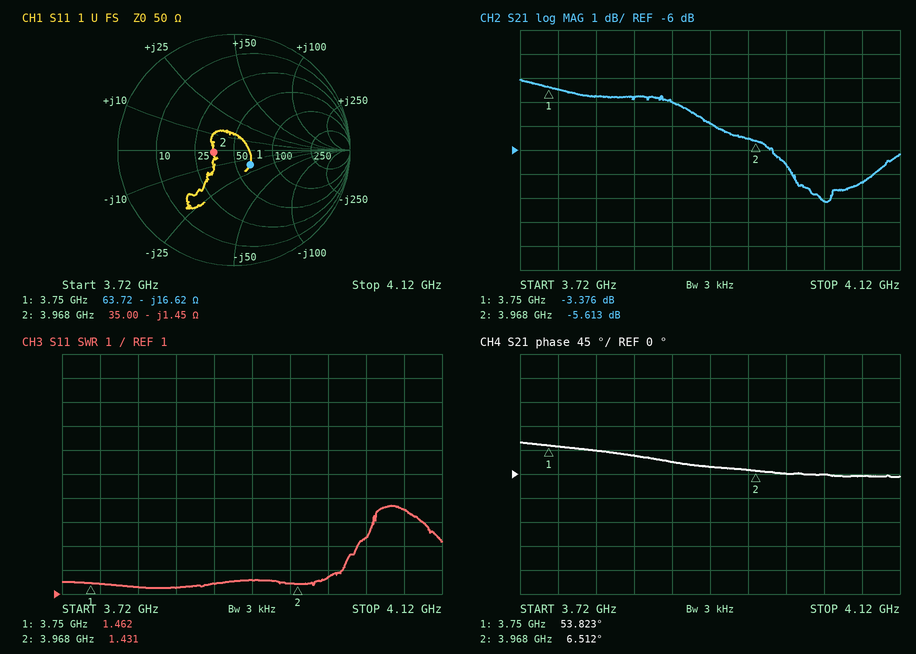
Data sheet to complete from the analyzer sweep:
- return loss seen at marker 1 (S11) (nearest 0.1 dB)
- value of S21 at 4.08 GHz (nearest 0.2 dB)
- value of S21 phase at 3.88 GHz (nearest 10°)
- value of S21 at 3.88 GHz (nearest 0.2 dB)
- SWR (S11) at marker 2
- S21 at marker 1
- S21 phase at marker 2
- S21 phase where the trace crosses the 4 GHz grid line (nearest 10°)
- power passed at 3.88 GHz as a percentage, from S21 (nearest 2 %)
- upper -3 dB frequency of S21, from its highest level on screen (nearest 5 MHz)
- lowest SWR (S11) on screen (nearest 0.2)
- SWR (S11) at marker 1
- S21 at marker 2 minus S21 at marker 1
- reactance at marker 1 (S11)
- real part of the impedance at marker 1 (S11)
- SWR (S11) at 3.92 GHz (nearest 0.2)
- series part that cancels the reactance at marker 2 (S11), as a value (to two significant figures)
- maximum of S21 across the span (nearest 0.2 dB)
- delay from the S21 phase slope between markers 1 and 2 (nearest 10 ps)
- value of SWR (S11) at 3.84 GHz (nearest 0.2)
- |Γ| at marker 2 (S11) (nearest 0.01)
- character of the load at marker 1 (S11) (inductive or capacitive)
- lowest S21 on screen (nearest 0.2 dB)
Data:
14.5 dB
-7.4 dB
20°
-4.0 dB
1.431
-3.376 dB
6.512°
0°
40 %
3.985 GHz
1.2
1.462
-2.237 dB
-16.62 Ω
63.72 Ω
1.6
58 pH
-3.0 dB
600 ps
1.2
0.18
capacitive
-8.2 dB
